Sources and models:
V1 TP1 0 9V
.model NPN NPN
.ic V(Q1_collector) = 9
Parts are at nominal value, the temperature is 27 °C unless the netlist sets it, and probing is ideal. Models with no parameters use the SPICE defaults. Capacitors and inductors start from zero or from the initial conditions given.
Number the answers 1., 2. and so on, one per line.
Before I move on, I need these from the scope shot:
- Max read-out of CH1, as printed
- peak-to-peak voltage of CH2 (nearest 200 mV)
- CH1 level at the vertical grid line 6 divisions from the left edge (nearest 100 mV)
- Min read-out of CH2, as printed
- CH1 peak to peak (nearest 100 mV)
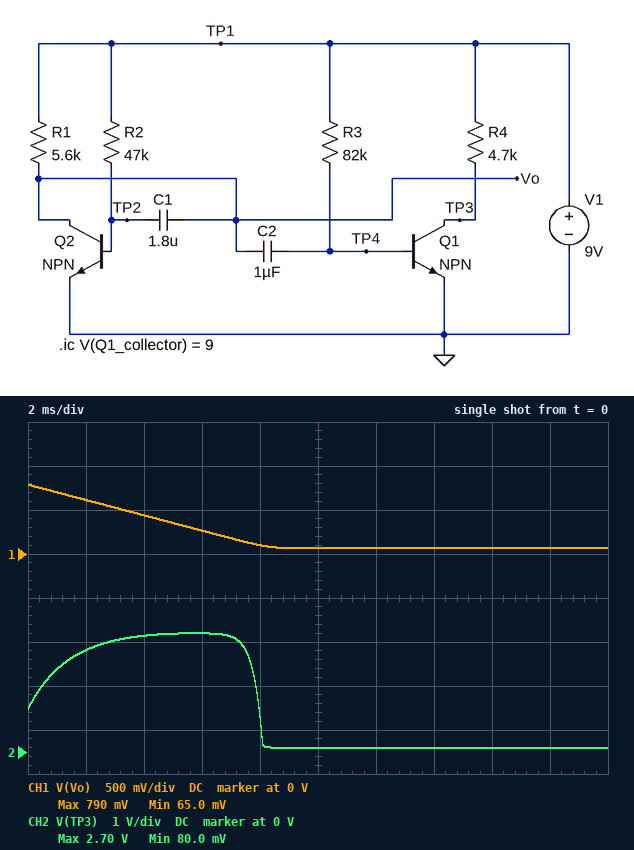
1. 790 mV
2. 2.6 V
3. 100 mV
4. 80.0 mV
5. 700 mV
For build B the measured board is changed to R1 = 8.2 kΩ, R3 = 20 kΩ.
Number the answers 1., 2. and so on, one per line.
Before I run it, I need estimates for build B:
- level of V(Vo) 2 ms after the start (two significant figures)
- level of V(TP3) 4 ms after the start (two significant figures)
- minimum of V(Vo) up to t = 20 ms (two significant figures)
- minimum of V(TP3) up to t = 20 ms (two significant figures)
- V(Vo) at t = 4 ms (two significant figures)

1. 600 mV
2. 55 mV
3. 56 mV
4. 50 mV
5. 420 mV
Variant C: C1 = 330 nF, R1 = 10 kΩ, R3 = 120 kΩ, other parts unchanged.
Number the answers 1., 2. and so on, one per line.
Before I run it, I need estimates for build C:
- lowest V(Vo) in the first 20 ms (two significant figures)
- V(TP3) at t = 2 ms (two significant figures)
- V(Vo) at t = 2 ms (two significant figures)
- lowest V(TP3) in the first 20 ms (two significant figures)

1. 52 mV
2. 9.0 V
3. 54 mV
4. 96 mV
